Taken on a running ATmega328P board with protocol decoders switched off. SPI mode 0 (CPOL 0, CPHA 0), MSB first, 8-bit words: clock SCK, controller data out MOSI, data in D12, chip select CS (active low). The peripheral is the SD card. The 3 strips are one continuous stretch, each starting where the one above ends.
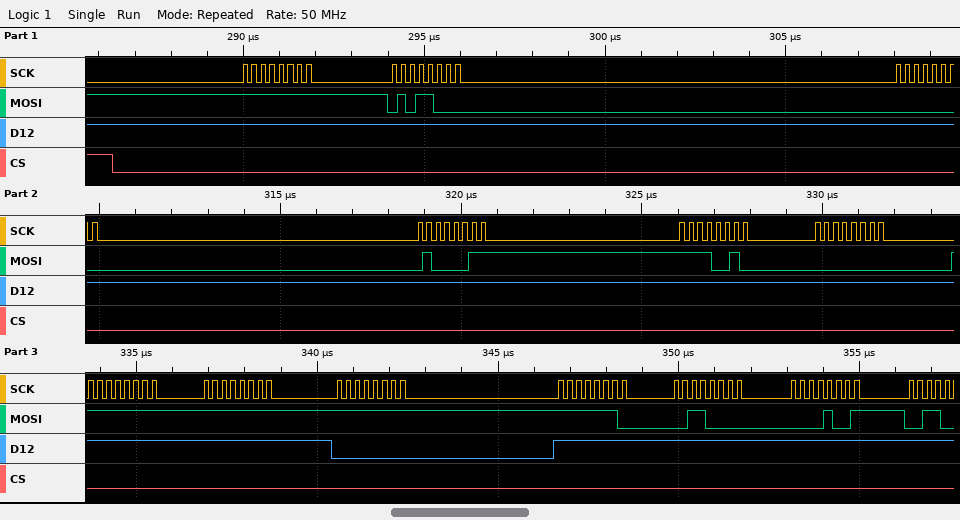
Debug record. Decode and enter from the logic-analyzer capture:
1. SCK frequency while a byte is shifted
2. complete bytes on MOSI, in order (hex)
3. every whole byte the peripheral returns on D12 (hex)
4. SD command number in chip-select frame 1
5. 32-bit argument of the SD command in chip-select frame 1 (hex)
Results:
4 MHz
0xFF 0x58 0x00 0x43 0xF2 0x00 0xFF 0xFF 0xFF 0xFE 0x30 0x09
0xFF 0xFF 0xFF 0xFF 0xFF 0xFF 0xFF 0xFF 0x00 0xFF 0xFF 0xFF
CMD24
0x0043F200
